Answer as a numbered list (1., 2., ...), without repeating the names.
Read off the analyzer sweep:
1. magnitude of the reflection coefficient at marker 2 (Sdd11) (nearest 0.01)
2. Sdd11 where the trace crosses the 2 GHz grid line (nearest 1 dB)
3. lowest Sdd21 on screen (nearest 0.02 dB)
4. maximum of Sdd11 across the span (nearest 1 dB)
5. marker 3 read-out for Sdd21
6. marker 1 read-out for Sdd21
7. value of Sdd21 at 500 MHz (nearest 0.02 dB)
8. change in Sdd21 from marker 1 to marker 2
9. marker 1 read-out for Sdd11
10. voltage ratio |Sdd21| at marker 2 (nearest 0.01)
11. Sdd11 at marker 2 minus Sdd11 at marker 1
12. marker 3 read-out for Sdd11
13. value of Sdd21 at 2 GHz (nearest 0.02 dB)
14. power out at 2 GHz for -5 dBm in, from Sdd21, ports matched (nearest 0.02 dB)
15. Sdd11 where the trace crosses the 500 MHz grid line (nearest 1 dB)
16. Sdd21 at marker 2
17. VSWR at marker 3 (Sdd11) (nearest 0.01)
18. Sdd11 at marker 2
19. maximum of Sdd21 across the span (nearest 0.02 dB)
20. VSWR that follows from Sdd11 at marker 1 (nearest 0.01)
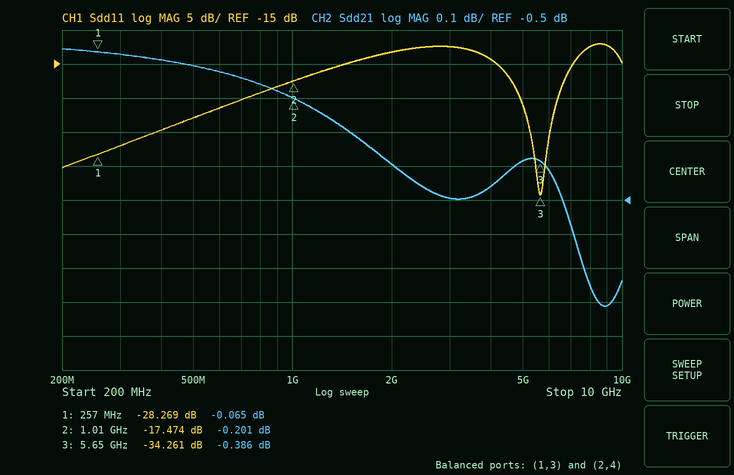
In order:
1. 0.13
2. -13 dB
3. -0.82 dB
4. -12 dB
5. -0.386 dB
6. -0.065 dB
7. -0.10 dB
8. -0.136 dB
9. -28.269 dB
10. 0.98
11. 10.795 dB
12. -34.261 dB
13. -0.40 dB
14. -5.40 dBm
15. -23 dB
16. -0.201 dB
17. 1.04
18. -17.474 dB
19. -0.06 dB
20. 1.08
